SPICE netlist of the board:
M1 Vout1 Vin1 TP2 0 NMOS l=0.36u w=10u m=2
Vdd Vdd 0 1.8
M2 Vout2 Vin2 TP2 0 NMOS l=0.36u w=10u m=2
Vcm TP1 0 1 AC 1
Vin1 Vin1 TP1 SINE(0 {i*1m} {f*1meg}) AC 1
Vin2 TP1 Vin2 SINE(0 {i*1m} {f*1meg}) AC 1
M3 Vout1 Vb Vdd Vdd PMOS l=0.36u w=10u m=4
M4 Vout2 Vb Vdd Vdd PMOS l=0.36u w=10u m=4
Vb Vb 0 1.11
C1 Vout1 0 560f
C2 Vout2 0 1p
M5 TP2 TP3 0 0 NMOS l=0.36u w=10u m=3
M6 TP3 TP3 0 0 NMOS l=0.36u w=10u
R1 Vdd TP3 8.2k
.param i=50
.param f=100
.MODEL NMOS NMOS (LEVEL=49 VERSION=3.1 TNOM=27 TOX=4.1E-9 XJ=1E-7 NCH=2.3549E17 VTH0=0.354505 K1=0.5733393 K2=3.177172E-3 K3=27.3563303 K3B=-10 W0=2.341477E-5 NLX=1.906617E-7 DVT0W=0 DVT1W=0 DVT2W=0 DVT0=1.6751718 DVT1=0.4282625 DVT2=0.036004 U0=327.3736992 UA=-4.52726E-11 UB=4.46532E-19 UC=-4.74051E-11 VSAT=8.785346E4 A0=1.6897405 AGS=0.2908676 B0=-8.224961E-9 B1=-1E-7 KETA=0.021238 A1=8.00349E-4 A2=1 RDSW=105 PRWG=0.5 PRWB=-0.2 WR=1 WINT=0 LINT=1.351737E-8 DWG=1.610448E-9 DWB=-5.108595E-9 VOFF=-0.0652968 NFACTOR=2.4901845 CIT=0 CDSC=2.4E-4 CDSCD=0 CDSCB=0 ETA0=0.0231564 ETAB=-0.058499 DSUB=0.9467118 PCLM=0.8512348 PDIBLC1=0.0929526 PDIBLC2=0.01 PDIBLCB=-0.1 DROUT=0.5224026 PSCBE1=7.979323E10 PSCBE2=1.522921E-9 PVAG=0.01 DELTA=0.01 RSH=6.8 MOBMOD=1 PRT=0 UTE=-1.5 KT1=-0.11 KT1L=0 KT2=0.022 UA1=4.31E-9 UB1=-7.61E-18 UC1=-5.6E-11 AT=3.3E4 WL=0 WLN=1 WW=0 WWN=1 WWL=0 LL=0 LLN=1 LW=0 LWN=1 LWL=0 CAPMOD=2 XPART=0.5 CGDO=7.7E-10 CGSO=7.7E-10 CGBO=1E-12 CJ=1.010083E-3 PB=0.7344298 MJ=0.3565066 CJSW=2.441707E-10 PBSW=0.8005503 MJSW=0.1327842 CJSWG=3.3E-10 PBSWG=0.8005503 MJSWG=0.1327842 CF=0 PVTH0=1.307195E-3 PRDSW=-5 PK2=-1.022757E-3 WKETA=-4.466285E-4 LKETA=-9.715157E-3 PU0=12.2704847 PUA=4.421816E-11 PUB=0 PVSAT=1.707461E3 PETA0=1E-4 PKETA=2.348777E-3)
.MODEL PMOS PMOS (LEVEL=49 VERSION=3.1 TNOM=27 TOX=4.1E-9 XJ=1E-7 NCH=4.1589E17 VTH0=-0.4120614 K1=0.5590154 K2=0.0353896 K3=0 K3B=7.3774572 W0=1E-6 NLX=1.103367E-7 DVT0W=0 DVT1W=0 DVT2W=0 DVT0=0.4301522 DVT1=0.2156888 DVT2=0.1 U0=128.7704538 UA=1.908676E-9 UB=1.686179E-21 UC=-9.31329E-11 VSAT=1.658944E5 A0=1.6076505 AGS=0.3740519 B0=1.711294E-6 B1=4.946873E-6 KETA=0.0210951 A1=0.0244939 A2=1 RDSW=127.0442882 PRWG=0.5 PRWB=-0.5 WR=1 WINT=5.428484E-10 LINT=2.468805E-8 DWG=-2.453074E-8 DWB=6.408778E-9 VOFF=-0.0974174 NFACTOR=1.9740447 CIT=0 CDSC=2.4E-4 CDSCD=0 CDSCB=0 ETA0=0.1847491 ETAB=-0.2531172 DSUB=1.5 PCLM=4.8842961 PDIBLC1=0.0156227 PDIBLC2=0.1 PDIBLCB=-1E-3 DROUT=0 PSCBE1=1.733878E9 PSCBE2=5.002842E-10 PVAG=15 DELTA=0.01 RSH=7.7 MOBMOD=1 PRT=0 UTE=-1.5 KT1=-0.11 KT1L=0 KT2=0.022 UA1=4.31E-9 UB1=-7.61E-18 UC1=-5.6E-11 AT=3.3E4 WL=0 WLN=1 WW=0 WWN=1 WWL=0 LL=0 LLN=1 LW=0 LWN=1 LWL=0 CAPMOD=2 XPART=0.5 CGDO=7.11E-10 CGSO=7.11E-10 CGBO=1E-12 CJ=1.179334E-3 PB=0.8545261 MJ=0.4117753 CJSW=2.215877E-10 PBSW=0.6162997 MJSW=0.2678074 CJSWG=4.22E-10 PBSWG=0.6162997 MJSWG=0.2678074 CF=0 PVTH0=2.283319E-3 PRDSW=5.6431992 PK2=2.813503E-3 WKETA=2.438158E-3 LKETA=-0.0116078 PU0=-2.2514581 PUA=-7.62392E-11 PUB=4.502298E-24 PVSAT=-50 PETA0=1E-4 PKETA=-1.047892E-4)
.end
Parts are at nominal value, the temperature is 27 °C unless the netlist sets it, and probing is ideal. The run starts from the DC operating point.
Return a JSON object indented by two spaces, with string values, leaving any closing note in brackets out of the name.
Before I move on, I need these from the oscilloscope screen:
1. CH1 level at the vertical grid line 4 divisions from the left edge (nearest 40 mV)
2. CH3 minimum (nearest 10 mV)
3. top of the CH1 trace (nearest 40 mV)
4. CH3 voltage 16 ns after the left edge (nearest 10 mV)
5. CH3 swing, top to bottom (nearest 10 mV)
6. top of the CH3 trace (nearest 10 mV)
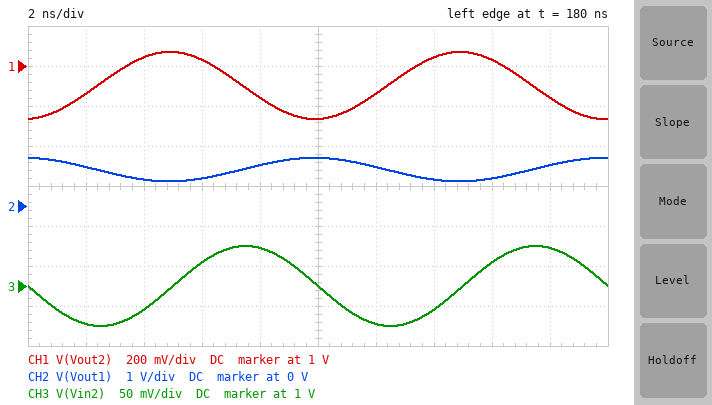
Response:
{
  "CH1 level at the vertical grid line 4 divisions from the left edge": "840 mV",
  "CH3 minimum": "950 mV",
  "top of the CH1 trace": "1.08 V",
  "CH3 voltage 16 ns after the left edge": "1.03 V",
  "CH3 swing, top to bottom": "100 mV",
  "top of the CH3 trace": "1.05 V"
}
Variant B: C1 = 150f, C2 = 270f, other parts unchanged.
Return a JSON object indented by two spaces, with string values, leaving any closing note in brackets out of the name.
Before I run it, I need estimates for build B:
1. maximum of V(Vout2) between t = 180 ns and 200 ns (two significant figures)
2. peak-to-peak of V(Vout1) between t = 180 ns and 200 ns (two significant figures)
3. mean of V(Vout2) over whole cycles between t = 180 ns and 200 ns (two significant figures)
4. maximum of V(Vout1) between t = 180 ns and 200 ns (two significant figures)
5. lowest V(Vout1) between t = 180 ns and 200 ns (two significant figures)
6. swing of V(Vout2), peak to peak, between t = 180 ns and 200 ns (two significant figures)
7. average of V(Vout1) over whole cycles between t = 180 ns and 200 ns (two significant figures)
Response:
{
  "maximum of V(Vout2) between t = 180 ns and 200 ns": "1.2 V",
  "peak-to-peak of V(Vout1) between t = 180 ns and 200 ns": "1.3 V",
  "mean of V(Vout2) over whole cycles between t = 180 ns and 200 ns": "770 mV",
  "maximum of V(Vout1) between t = 180 ns and 200 ns": "1.7 V",
  "lowest V(Vout1) between t = 180 ns and 200 ns": "320 mV",
  "swing of V(Vout2), peak to peak, between t = 180 ns and 200 ns": "810 mV",
  "average of V(Vout1) over whole cycles between t = 180 ns and 200 ns": "950 mV"
}
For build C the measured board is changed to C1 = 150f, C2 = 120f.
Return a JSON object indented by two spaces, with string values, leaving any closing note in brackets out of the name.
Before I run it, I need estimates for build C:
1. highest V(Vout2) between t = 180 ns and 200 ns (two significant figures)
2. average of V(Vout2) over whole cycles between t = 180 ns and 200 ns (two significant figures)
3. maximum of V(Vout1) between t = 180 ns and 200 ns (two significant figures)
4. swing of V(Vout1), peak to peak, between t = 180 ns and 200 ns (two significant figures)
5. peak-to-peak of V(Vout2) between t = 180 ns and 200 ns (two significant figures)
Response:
{
  "highest V(Vout2) between t = 180 ns and 200 ns": "1.6 V",
  "average of V(Vout2) over whole cycles between t = 180 ns and 200 ns": "930 mV",
  "maximum of V(Vout1) between t = 180 ns and 200 ns": "1.5 V",
  "swing of V(Vout1), peak to peak, between t = 180 ns and 200 ns": "1.2 V",
  "peak-to-peak of V(Vout2) between t = 180 ns and 200 ns": "1.3 V"
}
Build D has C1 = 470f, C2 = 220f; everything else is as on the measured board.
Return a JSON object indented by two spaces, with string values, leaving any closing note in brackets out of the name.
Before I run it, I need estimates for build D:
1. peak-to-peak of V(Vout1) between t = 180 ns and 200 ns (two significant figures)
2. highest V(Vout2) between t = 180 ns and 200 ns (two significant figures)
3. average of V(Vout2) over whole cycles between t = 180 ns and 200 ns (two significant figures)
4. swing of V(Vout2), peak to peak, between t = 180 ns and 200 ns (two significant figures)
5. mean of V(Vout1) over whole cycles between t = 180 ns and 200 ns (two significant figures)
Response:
{
  "peak-to-peak of V(Vout1) between t = 180 ns and 200 ns": "660 mV",
  "highest V(Vout2) between t = 180 ns and 200 ns": "1.6 V",
  "average of V(Vout2) over whole cycles between t = 180 ns and 200 ns": "970 mV",
  "swing of V(Vout2), peak to peak, between t = 180 ns and 200 ns": "1.2 V",
  "mean of V(Vout1) over whole cycles between t = 180 ns and 200 ns": "820 mV"
}
